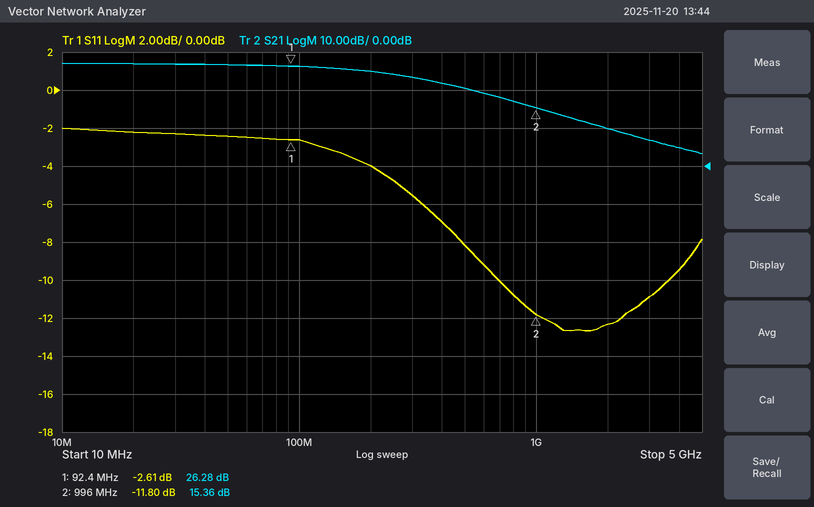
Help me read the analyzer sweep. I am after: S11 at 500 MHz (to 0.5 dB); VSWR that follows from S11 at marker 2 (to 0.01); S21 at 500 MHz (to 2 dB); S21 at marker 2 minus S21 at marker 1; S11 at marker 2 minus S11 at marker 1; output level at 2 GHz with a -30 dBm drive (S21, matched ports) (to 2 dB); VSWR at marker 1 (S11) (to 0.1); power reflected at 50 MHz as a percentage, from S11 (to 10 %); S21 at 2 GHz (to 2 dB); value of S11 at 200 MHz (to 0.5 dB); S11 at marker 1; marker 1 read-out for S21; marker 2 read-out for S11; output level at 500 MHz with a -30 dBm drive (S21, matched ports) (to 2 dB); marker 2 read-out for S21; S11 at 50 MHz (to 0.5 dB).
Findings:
-8.0 dB
1.69
20 dB
-10.92 dB
-9.19 dB
-20 dBm
6.7
60 %
10 dB
-4.0 dB
-2.61 dB
26.28 dB
-11.80 dB
-10 dBm
15.36 dB
-2.5 dB
